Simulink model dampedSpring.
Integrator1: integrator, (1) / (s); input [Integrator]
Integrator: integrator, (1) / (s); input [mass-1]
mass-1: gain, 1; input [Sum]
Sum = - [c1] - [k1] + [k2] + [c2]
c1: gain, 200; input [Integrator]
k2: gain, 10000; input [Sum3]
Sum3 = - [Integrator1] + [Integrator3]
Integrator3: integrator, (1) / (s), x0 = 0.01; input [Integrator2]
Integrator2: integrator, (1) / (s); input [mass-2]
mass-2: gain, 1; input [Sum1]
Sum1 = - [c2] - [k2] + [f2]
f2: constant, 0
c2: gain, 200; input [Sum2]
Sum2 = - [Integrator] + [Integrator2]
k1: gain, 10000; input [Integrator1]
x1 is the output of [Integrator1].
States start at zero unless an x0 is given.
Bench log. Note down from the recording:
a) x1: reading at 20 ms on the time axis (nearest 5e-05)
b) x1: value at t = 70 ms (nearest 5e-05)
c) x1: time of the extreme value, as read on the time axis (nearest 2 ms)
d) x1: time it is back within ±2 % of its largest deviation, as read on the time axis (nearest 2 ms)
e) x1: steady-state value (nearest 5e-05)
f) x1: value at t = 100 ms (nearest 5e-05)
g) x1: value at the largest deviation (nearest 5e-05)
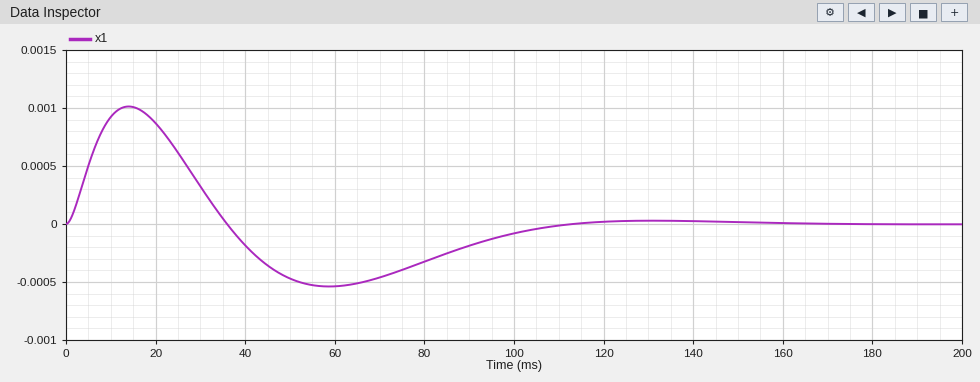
0.00085
-0.00045
14 ms
146 ms
0.00000
-0.00010
0.00100
